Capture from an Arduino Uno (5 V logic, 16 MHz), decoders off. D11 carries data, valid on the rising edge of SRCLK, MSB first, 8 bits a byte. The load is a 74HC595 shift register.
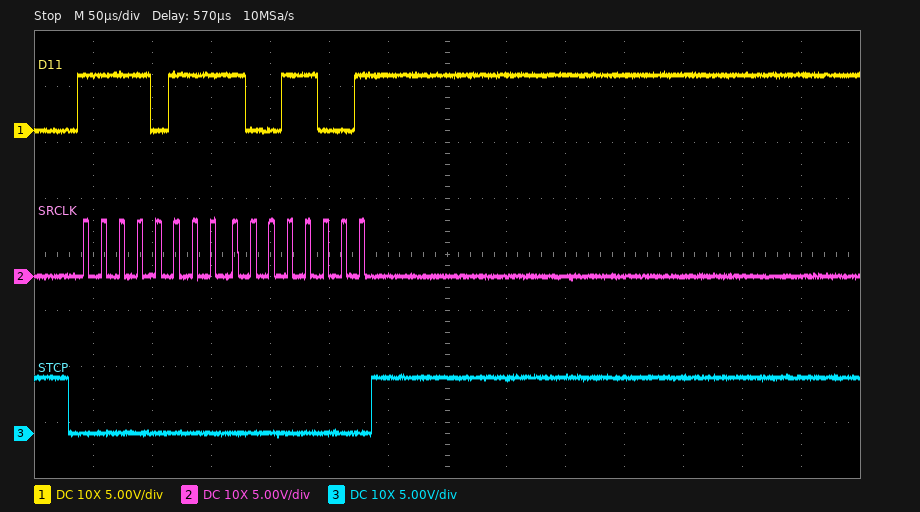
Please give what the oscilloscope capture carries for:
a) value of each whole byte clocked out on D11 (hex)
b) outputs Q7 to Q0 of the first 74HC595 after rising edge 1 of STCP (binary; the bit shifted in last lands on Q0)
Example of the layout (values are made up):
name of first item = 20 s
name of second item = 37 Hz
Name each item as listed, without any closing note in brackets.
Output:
value of each whole byte clocked out on D11 = F7 99
outputs Q7 to Q0 of the first 74HC595 after rising edge 1 of STCP = 10011001
